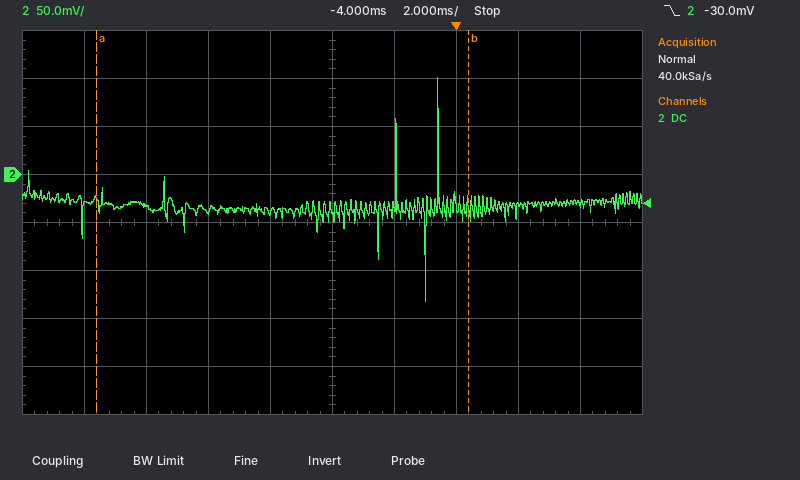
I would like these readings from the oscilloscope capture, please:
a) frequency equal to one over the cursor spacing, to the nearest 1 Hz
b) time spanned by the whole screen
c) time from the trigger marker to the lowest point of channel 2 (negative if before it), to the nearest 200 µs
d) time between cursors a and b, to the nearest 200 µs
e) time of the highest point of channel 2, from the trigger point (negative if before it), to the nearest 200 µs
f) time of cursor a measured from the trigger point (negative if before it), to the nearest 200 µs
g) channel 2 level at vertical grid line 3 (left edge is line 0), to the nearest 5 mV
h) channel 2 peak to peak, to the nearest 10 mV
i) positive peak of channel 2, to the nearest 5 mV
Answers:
83 Hz
20 ms
-1.0 ms
12.0 ms
-600 µs
-11.6 ms
-35 mV
230 mV
100 mV
